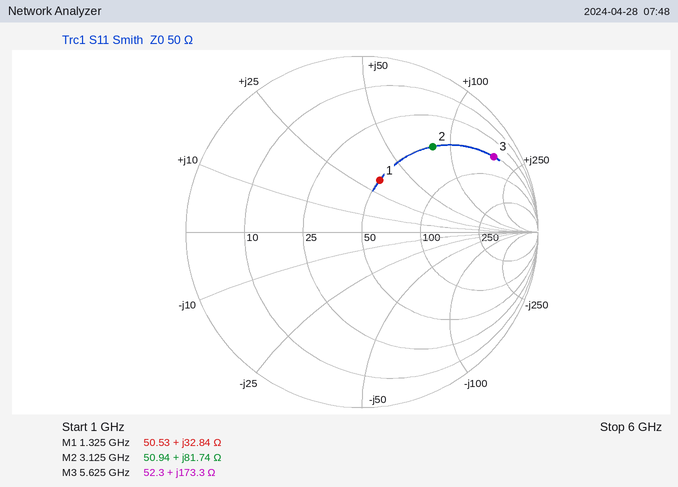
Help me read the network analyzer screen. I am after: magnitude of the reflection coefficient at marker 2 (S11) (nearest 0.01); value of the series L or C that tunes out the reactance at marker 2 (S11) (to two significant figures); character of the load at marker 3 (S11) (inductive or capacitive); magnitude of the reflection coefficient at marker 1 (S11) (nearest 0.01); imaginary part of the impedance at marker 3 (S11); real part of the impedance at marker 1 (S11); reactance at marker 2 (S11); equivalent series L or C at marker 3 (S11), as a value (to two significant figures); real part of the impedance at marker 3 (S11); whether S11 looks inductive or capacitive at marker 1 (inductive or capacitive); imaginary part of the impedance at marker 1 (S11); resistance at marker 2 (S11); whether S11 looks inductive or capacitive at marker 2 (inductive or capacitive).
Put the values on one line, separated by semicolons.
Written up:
0.63; 620 fF; inductive; 0.31; +173.3 Ω; 50.53 Ω; +81.74 Ω; 4.9 nH; 52.3 Ω; inductive; +32.84 Ω; 50.94 Ω; inductive
